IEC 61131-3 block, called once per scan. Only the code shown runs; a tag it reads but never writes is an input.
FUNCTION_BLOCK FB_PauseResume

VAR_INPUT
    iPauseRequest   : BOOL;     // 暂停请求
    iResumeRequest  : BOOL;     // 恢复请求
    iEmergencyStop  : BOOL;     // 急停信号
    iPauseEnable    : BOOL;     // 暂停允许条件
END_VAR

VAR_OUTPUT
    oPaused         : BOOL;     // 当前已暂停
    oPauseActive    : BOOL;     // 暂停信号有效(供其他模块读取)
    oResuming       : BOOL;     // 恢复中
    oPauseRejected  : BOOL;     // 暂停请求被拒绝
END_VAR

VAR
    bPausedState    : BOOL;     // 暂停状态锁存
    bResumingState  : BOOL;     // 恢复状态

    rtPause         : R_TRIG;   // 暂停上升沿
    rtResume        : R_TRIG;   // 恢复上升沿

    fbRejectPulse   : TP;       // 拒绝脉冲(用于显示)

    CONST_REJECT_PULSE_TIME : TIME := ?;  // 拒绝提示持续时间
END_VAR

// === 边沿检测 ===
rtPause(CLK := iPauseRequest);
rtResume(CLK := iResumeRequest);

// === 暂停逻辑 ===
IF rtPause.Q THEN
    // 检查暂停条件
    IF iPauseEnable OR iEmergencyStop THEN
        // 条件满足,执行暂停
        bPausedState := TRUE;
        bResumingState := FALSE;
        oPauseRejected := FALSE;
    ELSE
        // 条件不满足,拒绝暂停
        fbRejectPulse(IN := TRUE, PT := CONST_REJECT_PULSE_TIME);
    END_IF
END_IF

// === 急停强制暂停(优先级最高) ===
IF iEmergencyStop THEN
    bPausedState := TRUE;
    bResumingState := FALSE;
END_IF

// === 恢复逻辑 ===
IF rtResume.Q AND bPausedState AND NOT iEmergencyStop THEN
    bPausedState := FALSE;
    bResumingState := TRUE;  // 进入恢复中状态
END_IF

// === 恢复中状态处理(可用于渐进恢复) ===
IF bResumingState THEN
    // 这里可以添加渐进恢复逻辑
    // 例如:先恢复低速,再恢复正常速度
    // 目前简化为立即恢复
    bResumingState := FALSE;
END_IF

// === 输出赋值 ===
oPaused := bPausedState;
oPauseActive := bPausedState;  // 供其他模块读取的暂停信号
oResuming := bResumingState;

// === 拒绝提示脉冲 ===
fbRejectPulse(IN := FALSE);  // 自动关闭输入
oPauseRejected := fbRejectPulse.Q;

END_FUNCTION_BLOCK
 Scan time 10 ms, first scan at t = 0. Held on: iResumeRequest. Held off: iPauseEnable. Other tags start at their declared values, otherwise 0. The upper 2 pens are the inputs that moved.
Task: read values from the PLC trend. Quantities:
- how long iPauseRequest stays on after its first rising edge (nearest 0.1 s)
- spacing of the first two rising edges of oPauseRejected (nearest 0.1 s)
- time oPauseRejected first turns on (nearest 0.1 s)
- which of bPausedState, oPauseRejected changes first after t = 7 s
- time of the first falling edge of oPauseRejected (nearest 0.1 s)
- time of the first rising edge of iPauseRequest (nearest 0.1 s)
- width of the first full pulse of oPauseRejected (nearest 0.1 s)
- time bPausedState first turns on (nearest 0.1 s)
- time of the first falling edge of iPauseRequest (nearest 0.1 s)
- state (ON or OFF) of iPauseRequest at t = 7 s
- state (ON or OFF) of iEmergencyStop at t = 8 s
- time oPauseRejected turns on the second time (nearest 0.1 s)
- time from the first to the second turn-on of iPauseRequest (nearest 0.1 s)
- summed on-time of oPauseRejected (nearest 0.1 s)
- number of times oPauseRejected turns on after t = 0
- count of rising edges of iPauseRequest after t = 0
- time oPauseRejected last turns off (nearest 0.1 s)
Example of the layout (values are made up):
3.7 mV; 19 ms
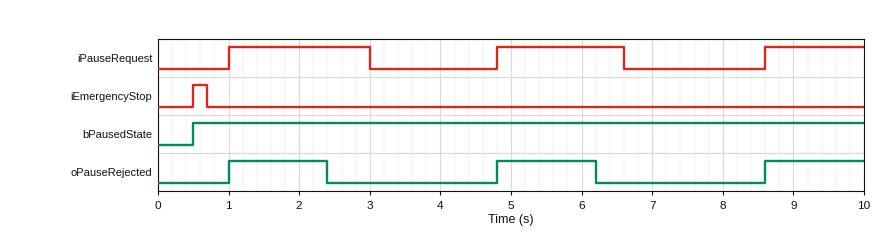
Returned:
2.0 s; 3.8 s; 1.0 s; oPauseRejected; 2.4 s; 1.0 s; 1.4 s; 0.5 s; 3.0 s; OFF; OFF; 4.8 s; 3.8 s; 4.2 s; 3; 3; 6.2 s
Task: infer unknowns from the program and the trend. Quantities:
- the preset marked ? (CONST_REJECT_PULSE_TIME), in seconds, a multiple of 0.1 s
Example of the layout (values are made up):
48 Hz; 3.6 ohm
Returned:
1.4 s
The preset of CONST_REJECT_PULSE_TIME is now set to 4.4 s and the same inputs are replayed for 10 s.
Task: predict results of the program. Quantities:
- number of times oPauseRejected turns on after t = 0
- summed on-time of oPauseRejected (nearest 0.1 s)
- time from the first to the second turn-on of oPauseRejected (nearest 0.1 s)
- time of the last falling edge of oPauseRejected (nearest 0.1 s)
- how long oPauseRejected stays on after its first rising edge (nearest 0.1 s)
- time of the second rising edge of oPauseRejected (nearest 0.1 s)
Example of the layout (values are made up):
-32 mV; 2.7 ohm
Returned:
2; 5.8 s; 7.6 s; 5.4 s; 4.4 s; 8.6 s
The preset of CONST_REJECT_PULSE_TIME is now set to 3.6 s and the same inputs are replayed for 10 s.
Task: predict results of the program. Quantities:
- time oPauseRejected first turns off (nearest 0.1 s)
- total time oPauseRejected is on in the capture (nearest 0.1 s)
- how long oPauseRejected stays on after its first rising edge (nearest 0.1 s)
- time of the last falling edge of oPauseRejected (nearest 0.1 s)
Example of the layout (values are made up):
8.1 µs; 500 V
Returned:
4.6 s; 8.6 s; 3.6 s; 8.4 s
